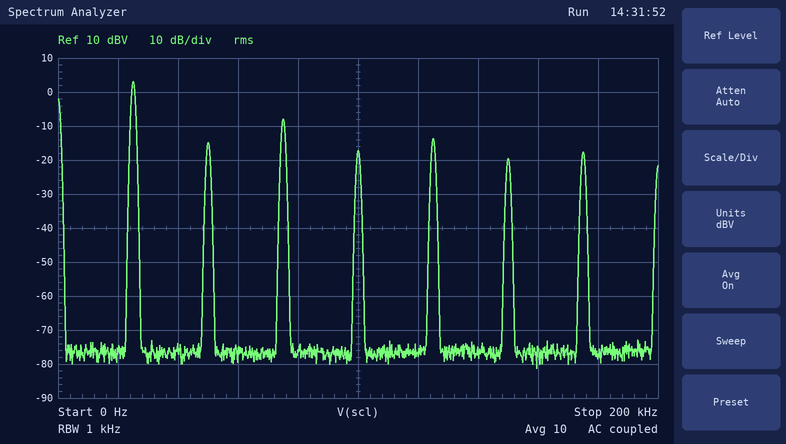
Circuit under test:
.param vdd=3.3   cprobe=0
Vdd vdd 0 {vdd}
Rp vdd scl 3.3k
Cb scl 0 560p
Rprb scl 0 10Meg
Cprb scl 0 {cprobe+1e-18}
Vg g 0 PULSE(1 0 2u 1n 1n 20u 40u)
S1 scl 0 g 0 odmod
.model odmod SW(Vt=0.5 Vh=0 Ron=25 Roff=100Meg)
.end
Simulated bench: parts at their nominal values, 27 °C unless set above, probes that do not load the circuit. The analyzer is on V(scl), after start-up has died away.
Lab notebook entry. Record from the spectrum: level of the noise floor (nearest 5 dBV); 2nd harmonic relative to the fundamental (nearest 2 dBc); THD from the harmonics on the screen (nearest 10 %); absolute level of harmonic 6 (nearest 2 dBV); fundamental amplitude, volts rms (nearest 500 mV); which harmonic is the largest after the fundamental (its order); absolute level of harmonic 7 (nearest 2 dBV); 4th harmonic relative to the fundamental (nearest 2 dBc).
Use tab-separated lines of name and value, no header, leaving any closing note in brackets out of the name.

level of the noise floor	-75 dBV
2nd harmonic relative to the fundamental	-18 dBc
THD from the harmonics on the screen	40 %
absolute level of harmonic 6	-20 dBV
fundamental amplitude, volts rms	1.5 V
which harmonic is the largest after the fundamental	3
absolute level of harmonic 7	-18 dBV
4th harmonic relative to the fundamental	-20 dBc
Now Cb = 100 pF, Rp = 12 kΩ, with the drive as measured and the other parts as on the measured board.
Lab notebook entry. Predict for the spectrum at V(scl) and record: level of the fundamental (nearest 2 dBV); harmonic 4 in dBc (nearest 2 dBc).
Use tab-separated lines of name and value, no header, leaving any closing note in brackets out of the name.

level of the fundamental	4 dBV
harmonic 4 in dBc	-22 dBc
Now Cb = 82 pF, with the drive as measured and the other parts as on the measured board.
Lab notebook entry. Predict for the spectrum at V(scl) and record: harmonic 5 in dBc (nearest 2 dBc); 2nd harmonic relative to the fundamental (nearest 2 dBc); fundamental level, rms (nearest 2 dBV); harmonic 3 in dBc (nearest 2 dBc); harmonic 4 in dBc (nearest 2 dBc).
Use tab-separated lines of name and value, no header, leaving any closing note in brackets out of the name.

harmonic 5 in dBc	-14 dBc
2nd harmonic relative to the fundamental	-34 dBc
fundamental level, rms	4 dBV
harmonic 3 in dBc	-10 dBc
harmonic 4 in dBc	-34 dBc
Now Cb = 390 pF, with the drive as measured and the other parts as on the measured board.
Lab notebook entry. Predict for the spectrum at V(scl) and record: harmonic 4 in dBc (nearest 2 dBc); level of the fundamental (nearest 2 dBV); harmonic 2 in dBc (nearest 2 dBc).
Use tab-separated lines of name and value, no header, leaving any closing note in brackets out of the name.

harmonic 4 in dBc	-22 dBc
level of the fundamental	4 dBV
harmonic 2 in dBc	-20 dBc
